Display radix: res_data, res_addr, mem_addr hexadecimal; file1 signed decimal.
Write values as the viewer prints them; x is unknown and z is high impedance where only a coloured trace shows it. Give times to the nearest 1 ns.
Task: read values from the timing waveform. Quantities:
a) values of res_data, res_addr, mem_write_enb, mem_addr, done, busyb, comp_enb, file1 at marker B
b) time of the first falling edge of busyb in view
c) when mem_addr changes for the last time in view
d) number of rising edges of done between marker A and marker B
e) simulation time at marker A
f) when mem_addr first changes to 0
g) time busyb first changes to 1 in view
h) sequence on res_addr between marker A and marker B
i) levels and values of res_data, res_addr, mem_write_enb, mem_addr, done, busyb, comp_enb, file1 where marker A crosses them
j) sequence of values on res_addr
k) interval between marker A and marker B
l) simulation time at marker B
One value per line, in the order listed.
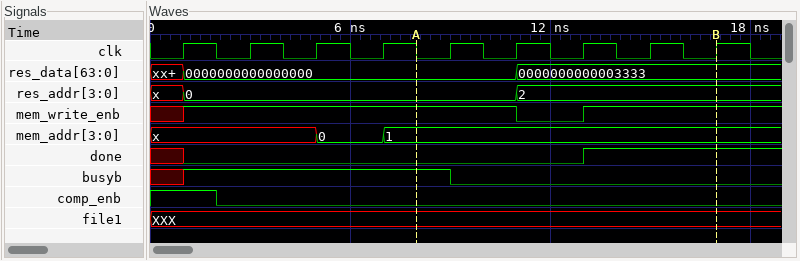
res_data=0000000000003333, res_addr=2, mem_write_enb=1, mem_addr=1, done=1, busyb=0, comp_enb=0, file1=XXX
9 ns
7 ns
1
8 ns
5 ns
1 ns
0, 2
res_data=0000000000000000, res_addr=0, mem_write_enb=1, mem_addr=1, done=0, busyb=1, comp_enb=0, file1=XXX
x, 0, 2
9 ns
17 ns
